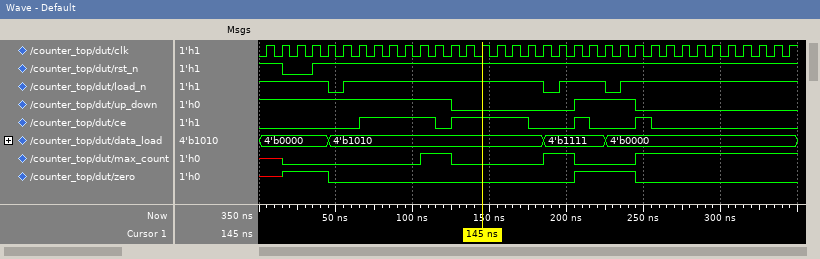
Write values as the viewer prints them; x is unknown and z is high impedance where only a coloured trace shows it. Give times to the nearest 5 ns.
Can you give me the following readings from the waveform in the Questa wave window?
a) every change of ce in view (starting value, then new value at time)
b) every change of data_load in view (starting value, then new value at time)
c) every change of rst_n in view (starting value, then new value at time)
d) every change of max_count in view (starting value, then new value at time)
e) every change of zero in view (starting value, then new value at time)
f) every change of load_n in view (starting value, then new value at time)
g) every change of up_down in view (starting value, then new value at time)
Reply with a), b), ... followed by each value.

a) 0, 1 at 65 ns, 0 at 115 ns, 1 at 125 ns, 0 at 175 ns, 1 at 205 ns, 0 at 215 ns, 1 at 245 ns, 0 at 255 ns
b) 4'b0000, 4'b1010 at 45 ns, 4'b1111 at 185 ns, 4'b0000 at 225 ns
c) 1, 0 at 15 ns, 1 at 35 ns
d) x, 0 at 15 ns, 1 at 105 ns, 0 at 125 ns, 1 at 185 ns, 0 at 205 ns, 1 at 245 ns
e) x, 1 at 15 ns, 0 at 45 ns, 1 at 205 ns, 0 at 245 ns
f) 1, 0 at 45 ns, 1 at 55 ns, 0 at 185 ns, 1 at 195 ns, 0 at 225 ns, 1 at 235 ns
g) 1, 0 at 125 ns, 1 at 205 ns, 0 at 245 ns
